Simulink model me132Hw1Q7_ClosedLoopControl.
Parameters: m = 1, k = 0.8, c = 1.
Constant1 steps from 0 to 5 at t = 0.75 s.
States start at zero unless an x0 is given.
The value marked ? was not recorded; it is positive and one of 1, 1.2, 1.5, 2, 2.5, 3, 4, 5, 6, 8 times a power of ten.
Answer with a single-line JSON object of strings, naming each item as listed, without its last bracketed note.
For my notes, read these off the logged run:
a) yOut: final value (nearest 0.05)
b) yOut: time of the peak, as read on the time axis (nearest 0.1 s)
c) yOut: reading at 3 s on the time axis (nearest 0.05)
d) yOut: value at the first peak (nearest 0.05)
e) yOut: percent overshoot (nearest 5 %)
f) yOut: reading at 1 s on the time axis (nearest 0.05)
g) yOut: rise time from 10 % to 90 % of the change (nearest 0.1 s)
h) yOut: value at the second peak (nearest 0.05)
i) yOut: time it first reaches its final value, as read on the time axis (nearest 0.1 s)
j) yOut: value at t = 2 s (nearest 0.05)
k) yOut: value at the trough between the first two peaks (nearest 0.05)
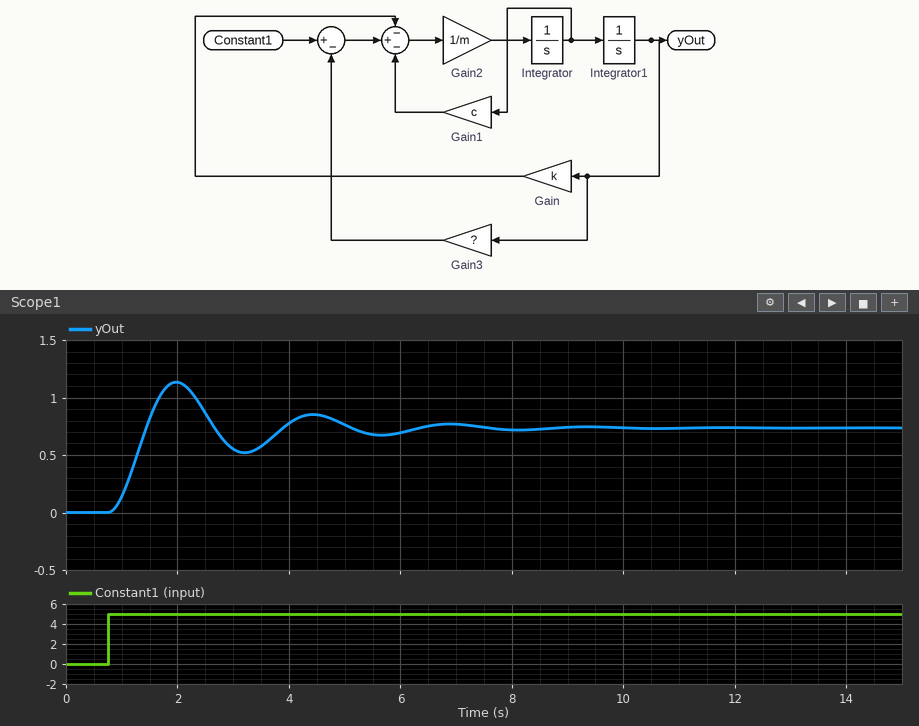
{"yOut: final value": "0.75", "yOut: time of the peak, as read on the time axis": "2.0 s", "yOut: reading at 3 s on the time axis": "0.55", "yOut: value at the first peak": "1.15", "yOut: percent overshoot": "55 %", "yOut: reading at 1 s on the time axis": "0.15", "yOut: rise time from 10 % to 90 % of the change": "0.5 s", "yOut: value at the second peak": "0.85", "yOut: time it first reaches its final value, as read on the time axis": "1.4 s", "yOut: value at t = 2 s": "1.15", "yOut: value at the trough between the first two peaks": "0.50"}
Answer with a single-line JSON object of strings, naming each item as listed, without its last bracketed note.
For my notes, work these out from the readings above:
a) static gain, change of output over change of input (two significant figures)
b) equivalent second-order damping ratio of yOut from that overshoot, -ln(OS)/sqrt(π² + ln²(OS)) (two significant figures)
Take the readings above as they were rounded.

{"static gain, change of output over change of input": "0.15", "equivalent second-order damping ratio of yOut from that overshoot, -ln(OS)/sqrt(π² + ln²(OS))": "0.19"}
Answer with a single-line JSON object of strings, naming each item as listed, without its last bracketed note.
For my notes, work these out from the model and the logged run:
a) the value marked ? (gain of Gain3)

{"the value marked ?": "6"}
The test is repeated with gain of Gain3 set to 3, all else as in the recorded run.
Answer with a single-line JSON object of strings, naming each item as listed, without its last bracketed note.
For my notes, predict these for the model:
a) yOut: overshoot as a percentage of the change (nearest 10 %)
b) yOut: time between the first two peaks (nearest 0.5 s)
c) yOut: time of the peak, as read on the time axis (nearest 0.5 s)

{"yOut: overshoot as a percentage of the change": "40 %", "yOut: time between the first two peaks": "3.5 s", "yOut: time of the peak, as read on the time axis": "2.5 s"}
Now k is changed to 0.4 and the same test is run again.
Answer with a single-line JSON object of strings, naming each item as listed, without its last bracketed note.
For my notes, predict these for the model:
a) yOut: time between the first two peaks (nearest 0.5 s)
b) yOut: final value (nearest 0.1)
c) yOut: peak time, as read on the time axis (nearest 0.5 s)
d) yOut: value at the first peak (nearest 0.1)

{"yOut: time between the first two peaks": "2.5 s", "yOut: final value": "0.8", "yOut: peak time, as read on the time axis": "2.0 s", "yOut: value at the first peak": "1.2"}
